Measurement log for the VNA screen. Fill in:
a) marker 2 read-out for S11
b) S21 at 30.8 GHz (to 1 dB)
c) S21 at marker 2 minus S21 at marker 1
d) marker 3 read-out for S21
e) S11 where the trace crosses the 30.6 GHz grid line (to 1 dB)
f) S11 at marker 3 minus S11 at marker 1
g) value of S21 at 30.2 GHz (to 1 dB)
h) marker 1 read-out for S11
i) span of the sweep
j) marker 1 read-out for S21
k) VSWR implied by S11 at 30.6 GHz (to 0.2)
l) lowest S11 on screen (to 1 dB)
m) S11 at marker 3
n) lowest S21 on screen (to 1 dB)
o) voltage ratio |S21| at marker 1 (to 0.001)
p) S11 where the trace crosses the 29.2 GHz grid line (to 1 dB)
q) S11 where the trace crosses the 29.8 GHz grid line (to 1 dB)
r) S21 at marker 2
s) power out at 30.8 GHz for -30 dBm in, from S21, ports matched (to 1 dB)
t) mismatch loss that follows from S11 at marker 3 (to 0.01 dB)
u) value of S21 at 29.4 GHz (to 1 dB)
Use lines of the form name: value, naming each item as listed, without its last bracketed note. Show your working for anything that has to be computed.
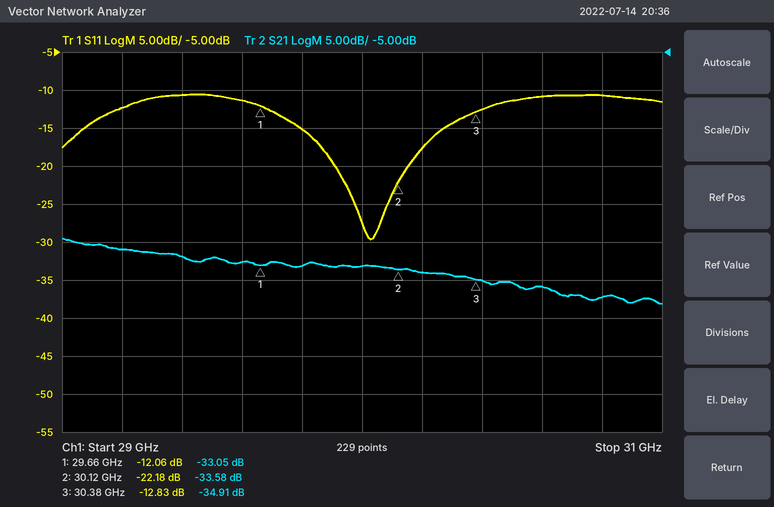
marker 2 read-out for S11: -22.18 dB
S21 at 30.8 GHz: -37 dB
S21 at marker 2 minus S21 at marker 1: -33.58 − (-33.05) = -0.53 dB
marker 3 read-out for S21: -34.91 dB
S11 where the trace crosses the 30.6 GHz grid line: -11 dB
S11 at marker 3 minus S11 at marker 1: -12.83 − (-12.06) = -0.77 dB
value of S21 at 30.2 GHz: -34 dB
marker 1 read-out for S11: -12.06 dB
span of the sweep: 2 GHz
marker 1 read-out for S21: -33.05 dB
VSWR implied by S11 at 30.6 GHz: |Γ| = 10^(-11/20) = 0.2818; VSWR = (1 + 0.2818)/(1 − 0.2818) ≈ 1.8
lowest S11 on screen: -30 dB
S11 at marker 3: -12.83 dB
lowest S21 on screen: -38 dB
voltage ratio |S21| at marker 1: 10^(-33.05/20) ≈ 0.022
S11 where the trace crosses the 29.2 GHz grid line: -12 dB
S11 where the trace crosses the 29.8 GHz grid line: -15 dB
S21 at marker 2: -33.58 dB
power out at 30.8 GHz for -30 dBm in, from S21, ports matched: -30 dBm + (-37 dB) = -67 dBm
mismatch loss that follows from S11 at marker 3: −10 log10(1 − 10^(-12.83/10)) ≈ 0.23 dB
value of S21 at 29.4 GHz: -32 dB
